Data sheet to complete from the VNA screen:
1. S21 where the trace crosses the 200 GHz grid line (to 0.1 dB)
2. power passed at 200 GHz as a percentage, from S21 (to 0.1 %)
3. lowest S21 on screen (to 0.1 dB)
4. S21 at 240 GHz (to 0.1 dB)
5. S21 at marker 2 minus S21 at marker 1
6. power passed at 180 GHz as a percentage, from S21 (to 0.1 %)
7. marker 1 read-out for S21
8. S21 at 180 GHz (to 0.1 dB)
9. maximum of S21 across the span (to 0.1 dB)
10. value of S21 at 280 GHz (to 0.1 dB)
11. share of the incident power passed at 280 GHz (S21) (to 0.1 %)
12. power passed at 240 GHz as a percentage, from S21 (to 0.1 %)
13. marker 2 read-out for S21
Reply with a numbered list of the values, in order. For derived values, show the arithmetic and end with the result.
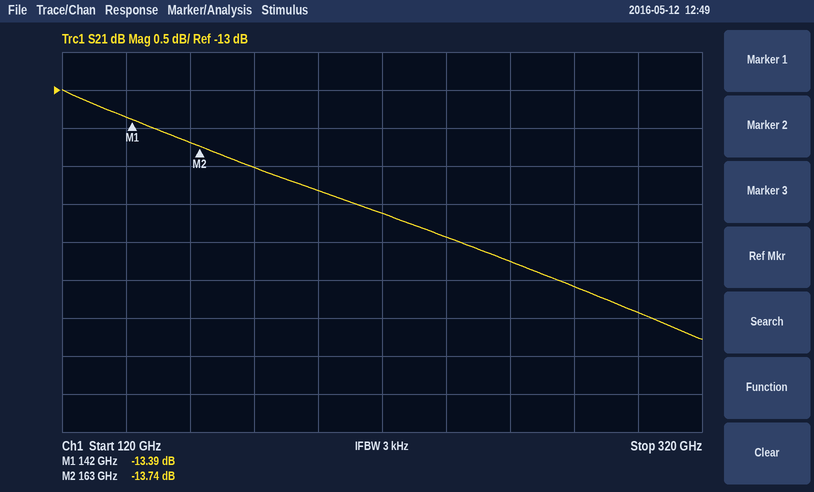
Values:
1. -14.3 dB
2. 10^(-14.3/10) ≈ 3.7 %
3. -16.3 dB
4. -14.9 dB
5. -13.74 − (-13.39) = -0.35 dB
6. 10^(-14/10) ≈ 4.0 %
7. -13.39 dB
8. -14.0 dB
9. -13.0 dB
10. -15.6 dB
11. 10^(-15.6/10) ≈ 2.8 %
12. 10^(-14.9/10) ≈ 3.2 %
13. -13.74 dB
